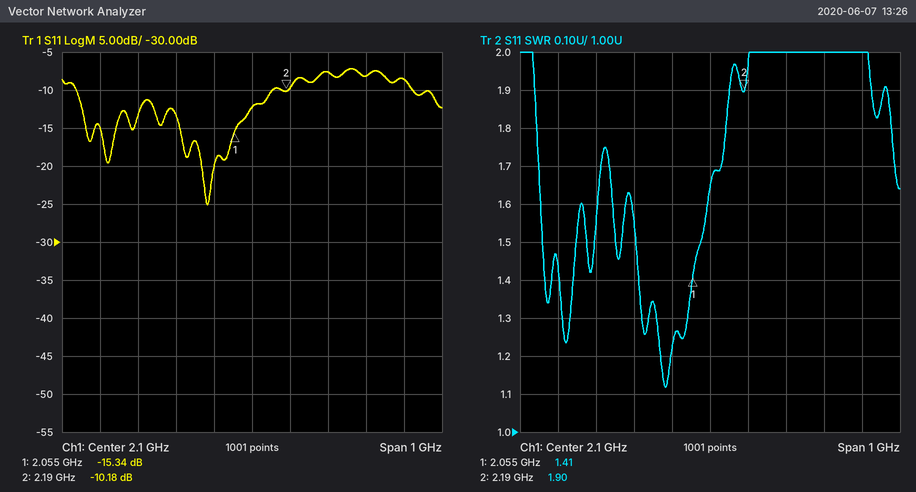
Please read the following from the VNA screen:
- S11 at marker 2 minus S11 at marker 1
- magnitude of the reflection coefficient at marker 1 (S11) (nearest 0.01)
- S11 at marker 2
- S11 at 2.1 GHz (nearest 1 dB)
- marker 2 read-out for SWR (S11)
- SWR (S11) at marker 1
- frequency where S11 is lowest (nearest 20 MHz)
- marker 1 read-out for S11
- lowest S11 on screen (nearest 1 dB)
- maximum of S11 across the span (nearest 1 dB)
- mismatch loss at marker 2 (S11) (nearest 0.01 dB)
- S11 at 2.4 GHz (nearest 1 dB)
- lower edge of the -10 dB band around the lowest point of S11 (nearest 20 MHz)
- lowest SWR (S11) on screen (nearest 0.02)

5.16 dB
0.17
-10.18 dB
-12 dB
1.90
1.41
1.98 GHz
-15.34 dB
-25 dB
-7 dB
0.44 dB
-8 dB
1.64 GHz
1.12
